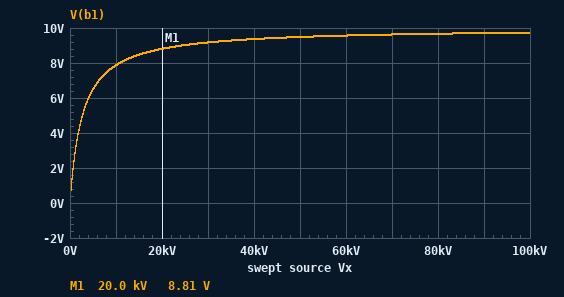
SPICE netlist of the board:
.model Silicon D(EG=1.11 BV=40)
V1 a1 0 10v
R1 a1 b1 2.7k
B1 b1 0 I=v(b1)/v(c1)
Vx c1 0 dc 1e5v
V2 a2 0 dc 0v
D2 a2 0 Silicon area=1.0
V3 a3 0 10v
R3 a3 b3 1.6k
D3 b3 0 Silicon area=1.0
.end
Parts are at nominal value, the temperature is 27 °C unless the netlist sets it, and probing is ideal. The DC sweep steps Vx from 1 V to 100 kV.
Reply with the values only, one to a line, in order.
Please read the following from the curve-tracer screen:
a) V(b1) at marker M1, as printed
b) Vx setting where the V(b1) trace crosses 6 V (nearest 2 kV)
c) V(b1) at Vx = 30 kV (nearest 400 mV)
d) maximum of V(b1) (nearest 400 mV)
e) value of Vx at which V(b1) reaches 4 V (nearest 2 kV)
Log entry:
8.81 V
4 kV
9.2 V
9.6 V
2 kV
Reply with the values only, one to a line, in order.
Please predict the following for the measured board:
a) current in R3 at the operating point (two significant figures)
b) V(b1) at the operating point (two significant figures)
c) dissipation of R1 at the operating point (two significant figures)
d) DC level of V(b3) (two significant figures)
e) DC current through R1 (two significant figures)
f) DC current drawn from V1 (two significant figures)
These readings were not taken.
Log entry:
5.8 mA
9.7 V
26 µW
700 mV
97 µA
97 µA
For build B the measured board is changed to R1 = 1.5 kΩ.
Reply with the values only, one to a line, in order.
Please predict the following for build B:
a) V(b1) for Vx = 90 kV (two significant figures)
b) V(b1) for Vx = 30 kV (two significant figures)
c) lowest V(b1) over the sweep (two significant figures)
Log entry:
9.8 V
9.5 V
6.7 mV
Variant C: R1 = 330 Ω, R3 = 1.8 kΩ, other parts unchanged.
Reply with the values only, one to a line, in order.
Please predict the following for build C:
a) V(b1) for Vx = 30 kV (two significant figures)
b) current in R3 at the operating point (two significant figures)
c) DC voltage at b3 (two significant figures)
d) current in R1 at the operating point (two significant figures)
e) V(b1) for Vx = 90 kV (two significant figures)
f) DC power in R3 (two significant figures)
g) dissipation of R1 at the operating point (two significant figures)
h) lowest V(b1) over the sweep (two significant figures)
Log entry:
9.9 V
5.2 mA
700 mV
100 µA
10 V
48 mW
3.3 µW
30 mV
